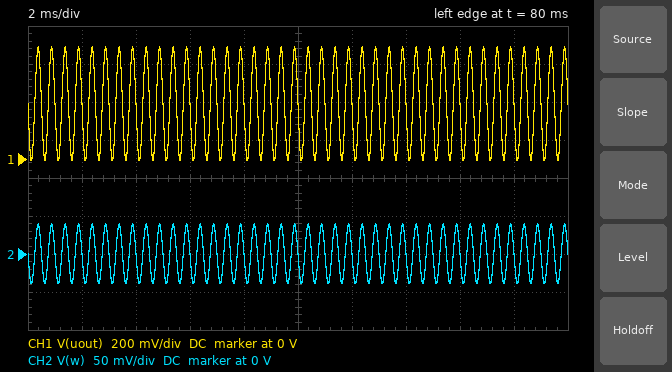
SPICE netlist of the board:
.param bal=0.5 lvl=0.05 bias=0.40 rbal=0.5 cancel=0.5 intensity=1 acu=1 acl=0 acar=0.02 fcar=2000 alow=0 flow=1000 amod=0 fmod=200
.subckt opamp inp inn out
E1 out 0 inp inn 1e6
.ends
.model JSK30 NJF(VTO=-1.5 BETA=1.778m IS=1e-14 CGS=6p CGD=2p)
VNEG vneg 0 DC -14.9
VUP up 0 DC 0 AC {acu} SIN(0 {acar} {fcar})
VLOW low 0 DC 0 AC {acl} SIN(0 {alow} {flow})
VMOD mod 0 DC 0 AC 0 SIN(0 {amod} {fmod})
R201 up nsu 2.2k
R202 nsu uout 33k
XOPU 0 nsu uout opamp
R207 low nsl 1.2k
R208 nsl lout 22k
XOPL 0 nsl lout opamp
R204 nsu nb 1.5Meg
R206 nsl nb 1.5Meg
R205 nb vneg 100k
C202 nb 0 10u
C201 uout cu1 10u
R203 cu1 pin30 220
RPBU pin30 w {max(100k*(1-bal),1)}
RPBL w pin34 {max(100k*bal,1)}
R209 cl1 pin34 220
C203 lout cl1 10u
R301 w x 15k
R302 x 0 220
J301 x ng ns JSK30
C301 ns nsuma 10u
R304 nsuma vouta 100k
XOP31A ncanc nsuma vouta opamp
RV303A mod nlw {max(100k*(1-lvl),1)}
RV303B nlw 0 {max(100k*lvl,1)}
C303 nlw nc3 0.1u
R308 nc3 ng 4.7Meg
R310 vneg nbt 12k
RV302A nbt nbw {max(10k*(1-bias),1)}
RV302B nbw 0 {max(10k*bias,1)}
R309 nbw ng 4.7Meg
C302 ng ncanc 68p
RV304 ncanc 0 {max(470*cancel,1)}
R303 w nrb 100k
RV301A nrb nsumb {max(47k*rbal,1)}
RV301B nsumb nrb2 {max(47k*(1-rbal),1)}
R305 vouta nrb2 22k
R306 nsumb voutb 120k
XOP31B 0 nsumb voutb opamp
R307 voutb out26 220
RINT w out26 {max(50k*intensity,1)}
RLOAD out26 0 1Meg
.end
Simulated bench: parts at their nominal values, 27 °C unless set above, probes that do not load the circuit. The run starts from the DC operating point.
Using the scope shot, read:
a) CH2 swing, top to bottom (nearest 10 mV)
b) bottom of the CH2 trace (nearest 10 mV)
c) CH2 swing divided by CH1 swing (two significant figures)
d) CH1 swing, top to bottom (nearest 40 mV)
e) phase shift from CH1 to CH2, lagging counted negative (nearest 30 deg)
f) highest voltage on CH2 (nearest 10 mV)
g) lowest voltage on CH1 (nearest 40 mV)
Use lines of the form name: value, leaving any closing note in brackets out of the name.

CH2 swing, top to bottom: 80 mV
bottom of the CH2 trace: -40 mV
CH2 swing divided by CH1 swing: 0.13
CH1 swing, top to bottom: 600 mV
phase shift from CH1 to CH2, lagging counted negative: 0 deg
highest voltage on CH2: 40 mV
lowest voltage on CH1: 0 V
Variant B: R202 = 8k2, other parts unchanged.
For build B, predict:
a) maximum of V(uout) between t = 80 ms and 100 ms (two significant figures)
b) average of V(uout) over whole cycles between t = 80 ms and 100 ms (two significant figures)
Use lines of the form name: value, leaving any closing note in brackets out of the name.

maximum of V(uout) between t = 80 ms and 100 ms: 150 mV
average of V(uout) over whole cycles between t = 80 ms and 100 ms: 72 mV
